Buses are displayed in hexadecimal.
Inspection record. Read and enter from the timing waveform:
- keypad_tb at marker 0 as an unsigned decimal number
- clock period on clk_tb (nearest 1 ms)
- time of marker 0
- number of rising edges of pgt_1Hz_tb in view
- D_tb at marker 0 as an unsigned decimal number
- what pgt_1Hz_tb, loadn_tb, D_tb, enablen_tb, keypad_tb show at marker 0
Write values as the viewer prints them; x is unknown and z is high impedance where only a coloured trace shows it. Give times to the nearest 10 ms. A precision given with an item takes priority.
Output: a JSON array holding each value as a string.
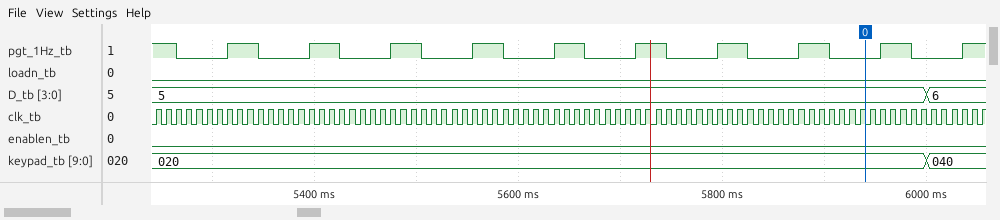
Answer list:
["32", "10 ms", "5940 ms", "10", "5", "pgt_1Hz_tb=0, loadn_tb=0, D_tb=5, enablen_tb=0, keypad_tb=020"]
